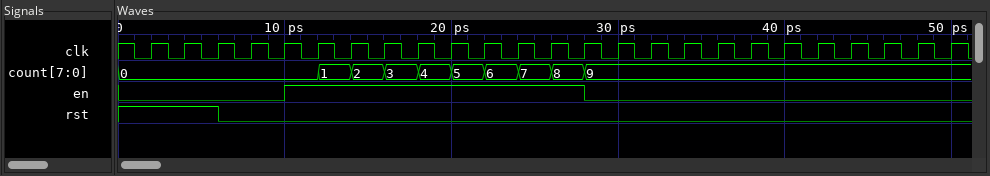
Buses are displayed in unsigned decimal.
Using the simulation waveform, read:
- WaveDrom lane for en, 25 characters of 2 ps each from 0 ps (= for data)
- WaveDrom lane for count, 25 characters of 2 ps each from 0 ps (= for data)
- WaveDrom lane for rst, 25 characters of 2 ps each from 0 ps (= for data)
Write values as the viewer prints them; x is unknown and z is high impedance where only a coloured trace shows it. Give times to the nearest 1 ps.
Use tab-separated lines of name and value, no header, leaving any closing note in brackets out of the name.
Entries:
WaveDrom lane for en, 25 characters of 2 ps each from 0 ps	{name: 'en', wave: '0....1........0..........'}
WaveDrom lane for count, 25 characters of 2 ps each from 0 ps	{name: 'count', wave: '=.....=========..........', data: '0 1 2 3 4 5 6 7 8 9'}
WaveDrom lane for rst, 25 characters of 2 ps each from 0 ps	{name: 'rst', wave: '1..0.....................'}
